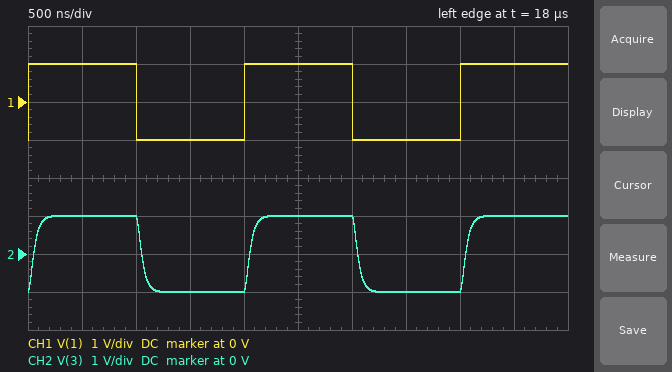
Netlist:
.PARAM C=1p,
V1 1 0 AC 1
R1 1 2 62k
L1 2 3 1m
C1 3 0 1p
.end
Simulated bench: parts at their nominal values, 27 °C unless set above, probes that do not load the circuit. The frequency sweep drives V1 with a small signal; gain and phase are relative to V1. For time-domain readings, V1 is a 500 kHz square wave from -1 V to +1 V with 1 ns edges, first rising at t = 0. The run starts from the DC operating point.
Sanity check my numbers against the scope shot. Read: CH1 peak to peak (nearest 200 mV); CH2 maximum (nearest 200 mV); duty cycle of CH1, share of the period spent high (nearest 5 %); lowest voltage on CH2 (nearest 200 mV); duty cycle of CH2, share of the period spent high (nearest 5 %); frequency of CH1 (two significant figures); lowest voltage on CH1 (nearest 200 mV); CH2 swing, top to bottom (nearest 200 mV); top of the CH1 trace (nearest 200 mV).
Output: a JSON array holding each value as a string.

["2.0 V", "1.0 V", "50 %", "-1.0 V", "50 %", "500 kHz", "-1.0 V", "2.0 V", "1.0 V"]
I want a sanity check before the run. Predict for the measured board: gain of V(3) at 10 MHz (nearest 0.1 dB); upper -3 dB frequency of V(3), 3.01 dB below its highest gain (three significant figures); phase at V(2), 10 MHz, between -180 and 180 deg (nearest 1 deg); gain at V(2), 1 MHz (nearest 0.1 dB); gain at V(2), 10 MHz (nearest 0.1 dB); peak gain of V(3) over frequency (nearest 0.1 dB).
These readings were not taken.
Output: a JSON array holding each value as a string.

["-13.8 dB", "3.33 MHz", "53 deg", "-0.7 dB", "-4.4 dB", "0 dB"]
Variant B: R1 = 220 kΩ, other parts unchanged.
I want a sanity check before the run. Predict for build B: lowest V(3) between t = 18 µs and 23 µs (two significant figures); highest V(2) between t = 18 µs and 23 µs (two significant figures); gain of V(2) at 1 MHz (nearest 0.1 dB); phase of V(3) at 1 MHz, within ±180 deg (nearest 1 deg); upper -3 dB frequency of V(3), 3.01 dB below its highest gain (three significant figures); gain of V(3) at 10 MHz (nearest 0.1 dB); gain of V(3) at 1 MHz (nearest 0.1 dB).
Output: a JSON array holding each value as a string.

["-980 mV", "980 mV", "-4.9 dB", "-55 deg", "739 kHz", "-23.0 dB", "-4.5 dB"]
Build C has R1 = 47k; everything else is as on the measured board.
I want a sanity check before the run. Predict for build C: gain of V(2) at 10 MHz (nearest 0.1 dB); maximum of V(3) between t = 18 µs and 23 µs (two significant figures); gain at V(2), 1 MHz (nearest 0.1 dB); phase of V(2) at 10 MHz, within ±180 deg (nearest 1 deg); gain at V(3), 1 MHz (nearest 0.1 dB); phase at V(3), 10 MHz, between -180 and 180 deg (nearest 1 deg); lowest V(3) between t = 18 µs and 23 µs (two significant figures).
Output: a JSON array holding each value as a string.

["-3.0 dB", "1.1 V", "-0.4 dB", "45 deg", "0 dB", "-135 deg", "-1.1 V"]
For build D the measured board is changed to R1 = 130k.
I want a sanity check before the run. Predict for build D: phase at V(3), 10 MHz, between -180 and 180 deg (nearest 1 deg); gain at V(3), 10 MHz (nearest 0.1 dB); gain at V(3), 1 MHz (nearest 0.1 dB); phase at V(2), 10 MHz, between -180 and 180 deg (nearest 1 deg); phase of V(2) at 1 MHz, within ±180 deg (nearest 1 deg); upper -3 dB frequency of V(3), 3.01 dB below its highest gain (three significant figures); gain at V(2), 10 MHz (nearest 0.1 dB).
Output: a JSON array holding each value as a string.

["-110 deg", "-18.8 dB", "-2.0 dB", "70 deg", "-40 deg", "1.30 MHz", "-9.4 dB"]
